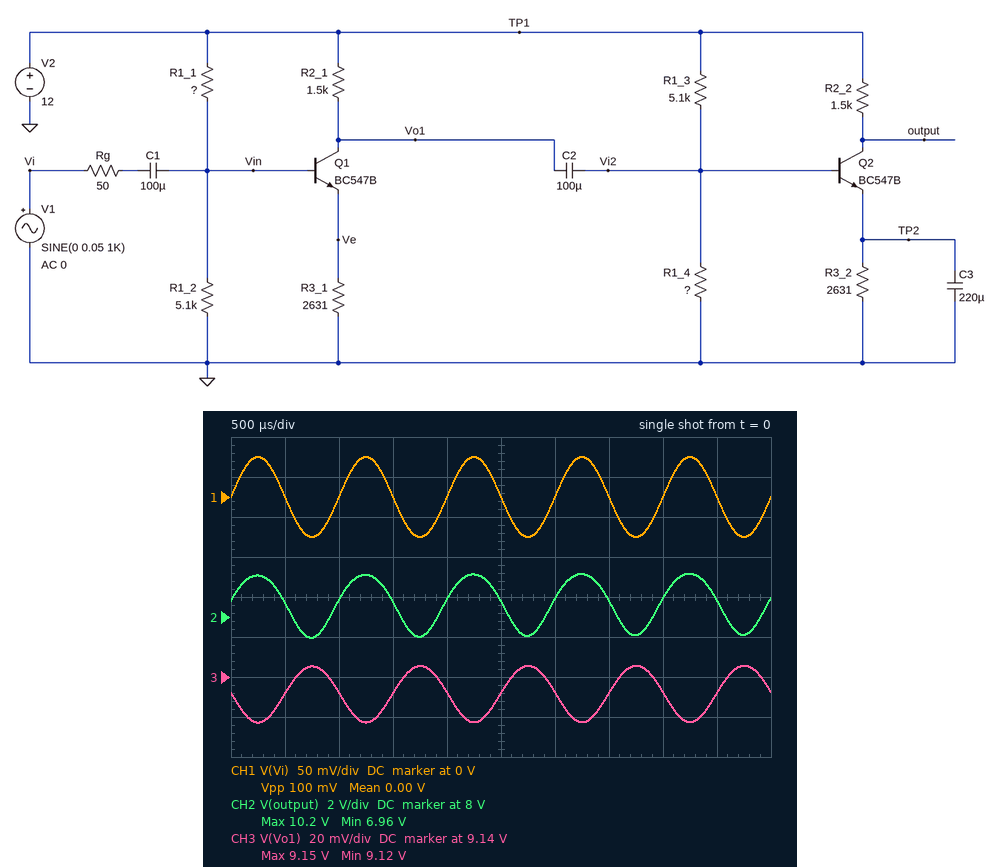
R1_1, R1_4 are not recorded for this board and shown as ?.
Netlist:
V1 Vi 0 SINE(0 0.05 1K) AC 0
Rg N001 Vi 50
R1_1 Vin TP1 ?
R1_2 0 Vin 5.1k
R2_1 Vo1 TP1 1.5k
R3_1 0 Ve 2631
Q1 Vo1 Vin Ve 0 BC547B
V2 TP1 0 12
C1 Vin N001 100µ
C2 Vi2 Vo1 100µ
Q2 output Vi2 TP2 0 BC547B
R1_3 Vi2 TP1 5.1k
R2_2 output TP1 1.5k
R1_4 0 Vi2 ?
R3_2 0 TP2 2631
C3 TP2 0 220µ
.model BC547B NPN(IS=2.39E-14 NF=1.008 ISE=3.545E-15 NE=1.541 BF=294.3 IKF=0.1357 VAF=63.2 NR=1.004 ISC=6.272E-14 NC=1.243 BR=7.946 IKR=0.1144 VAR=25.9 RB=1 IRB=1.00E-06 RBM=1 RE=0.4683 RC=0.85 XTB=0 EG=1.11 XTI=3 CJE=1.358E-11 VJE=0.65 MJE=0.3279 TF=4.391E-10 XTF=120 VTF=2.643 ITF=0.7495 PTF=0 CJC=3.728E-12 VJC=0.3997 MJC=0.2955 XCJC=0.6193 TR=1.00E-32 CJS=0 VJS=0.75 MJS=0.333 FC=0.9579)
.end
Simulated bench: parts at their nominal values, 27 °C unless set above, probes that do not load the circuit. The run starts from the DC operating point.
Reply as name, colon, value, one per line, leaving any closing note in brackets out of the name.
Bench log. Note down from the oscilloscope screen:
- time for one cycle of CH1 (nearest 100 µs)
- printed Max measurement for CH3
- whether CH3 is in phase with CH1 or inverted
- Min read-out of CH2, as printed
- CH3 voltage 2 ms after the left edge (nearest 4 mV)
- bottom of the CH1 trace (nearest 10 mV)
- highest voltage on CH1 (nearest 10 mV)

time for one cycle of CH1: 1.0 ms
printed Max measurement for CH3: 9.15 V
whether CH3 is in phase with CH1 or inverted: inverted
Min read-out of CH2, as printed: 6.96 V
CH3 voltage 2 ms after the left edge: 9.132 V
bottom of the CH1 trace: -50 mV
highest voltage on CH1: 50 mV
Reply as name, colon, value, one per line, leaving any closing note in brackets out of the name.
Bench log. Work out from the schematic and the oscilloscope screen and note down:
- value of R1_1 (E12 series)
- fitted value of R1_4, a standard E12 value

value of R1_1: 5.6 kΩ
fitted value of R1_4, a standard E12 value: 5.6 kΩ
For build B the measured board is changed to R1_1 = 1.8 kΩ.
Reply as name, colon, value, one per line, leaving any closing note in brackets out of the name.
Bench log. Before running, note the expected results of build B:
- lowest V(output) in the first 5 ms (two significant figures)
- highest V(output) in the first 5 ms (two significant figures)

lowest V(output) in the first 5 ms: 5.7 V
highest V(output) in the first 5 ms: 11 V
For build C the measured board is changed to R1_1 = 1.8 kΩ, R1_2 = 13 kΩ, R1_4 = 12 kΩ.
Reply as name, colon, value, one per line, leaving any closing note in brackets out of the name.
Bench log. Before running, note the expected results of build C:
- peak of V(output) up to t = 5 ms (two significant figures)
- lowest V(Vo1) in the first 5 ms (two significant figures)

peak of V(output) up to t = 5 ms: 11 V
lowest V(Vo1) in the first 5 ms: 8.4 V
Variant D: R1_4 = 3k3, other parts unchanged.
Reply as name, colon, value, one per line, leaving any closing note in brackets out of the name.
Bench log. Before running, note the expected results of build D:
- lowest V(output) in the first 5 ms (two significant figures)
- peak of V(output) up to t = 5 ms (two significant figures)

lowest V(output) in the first 5 ms: 8.3 V
peak of V(output) up to t = 5 ms: 11 V
